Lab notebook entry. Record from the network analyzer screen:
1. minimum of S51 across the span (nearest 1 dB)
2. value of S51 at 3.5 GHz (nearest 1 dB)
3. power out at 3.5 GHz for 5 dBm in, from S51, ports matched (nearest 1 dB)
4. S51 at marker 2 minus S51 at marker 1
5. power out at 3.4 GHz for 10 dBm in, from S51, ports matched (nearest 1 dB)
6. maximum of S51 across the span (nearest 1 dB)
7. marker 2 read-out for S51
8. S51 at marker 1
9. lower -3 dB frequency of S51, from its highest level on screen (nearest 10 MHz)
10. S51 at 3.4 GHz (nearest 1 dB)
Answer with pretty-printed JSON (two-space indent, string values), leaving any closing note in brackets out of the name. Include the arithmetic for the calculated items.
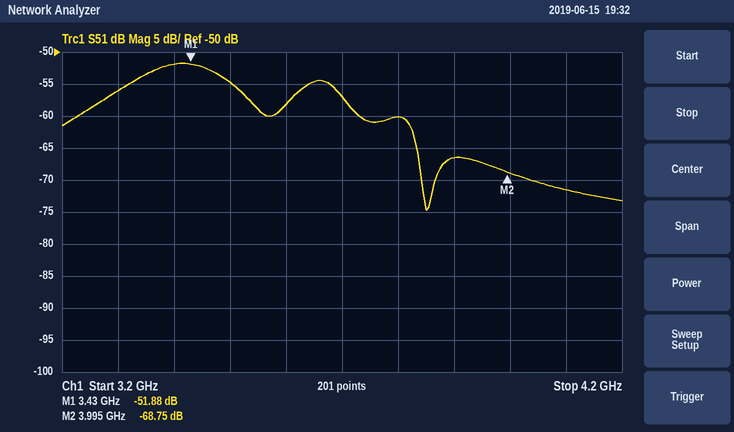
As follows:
{
  "minimum of S51 across the span": "-75 dB",
  "value of S51 at 3.5 GHz": "-55 dB",
  "power out at 3.5 GHz for 5 dBm in, from S51, ports matched": "5 dBm + (-55 dB) = -50 dBm",
  "S51 at marker 2 minus S51 at marker 1": "-68.75 − (-51.88) = -16.87 dB",
  "power out at 3.4 GHz for 10 dBm in, from S51, ports matched": "10 dBm + (-52 dB) = -42 dBm",
  "maximum of S51 across the span": "-52 dB",
  "marker 2 read-out for S51": "-68.75 dB",
  "S51 at marker 1": "-51.88 dB",
  "lower -3 dB frequency of S51, from its highest level on screen": "3.32 GHz",
  "S51 at 3.4 GHz": "-52 dB"
}
